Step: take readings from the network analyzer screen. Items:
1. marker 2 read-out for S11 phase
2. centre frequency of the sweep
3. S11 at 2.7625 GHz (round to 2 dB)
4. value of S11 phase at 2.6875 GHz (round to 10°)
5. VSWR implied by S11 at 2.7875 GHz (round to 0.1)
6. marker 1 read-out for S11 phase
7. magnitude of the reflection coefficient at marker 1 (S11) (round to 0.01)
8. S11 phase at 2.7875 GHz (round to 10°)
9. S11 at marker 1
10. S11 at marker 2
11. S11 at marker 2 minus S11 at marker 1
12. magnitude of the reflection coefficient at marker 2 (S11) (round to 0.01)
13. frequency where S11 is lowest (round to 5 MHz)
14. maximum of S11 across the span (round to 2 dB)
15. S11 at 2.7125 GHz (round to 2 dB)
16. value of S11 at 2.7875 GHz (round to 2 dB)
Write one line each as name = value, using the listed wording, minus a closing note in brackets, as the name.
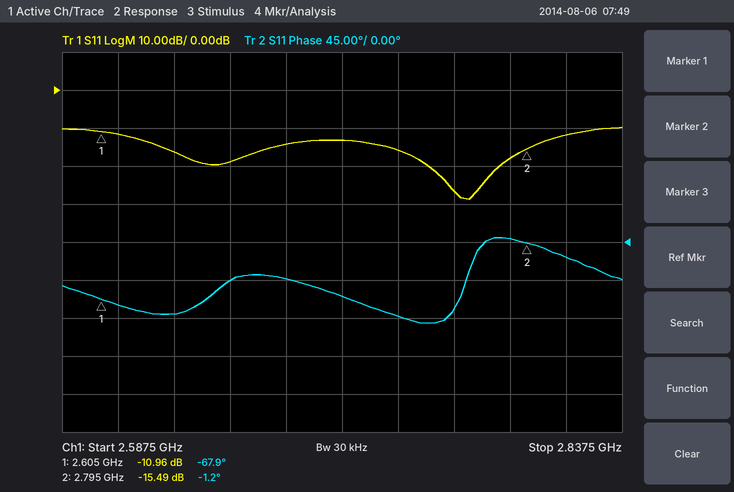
marker 2 read-out for S11 phase = -1.2°
centre frequency of the sweep = 2.7125 GHz
S11 at 2.7625 GHz = -26 dB
value of S11 phase at 2.6875 GHz = -40°
VSWR implied by S11 at 2.7875 GHz = 1.3
marker 1 read-out for S11 phase = -67.9°
magnitude of the reflection coefficient at marker 1 (S11) = 0.28
S11 phase at 2.7875 GHz = 0°
S11 at marker 1 = -10.96 dB
S11 at marker 2 = -15.49 dB
S11 at marker 2 minus S11 at marker 1 = -4.53 dB
magnitude of the reflection coefficient at marker 2 (S11) = 0.17
frequency where S11 is lowest = 2.770 GHz
maximum of S11 across the span = -10 dB
S11 at 2.7125 GHz = -14 dB
value of S11 at 2.7875 GHz = -18 dB
